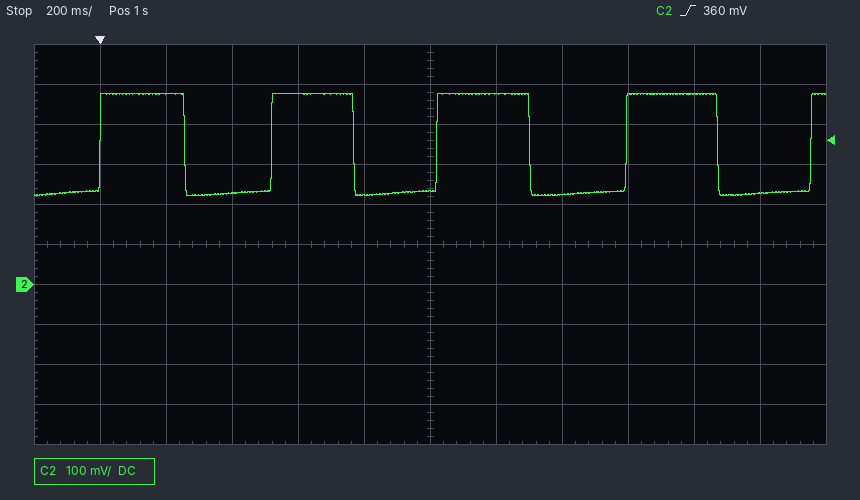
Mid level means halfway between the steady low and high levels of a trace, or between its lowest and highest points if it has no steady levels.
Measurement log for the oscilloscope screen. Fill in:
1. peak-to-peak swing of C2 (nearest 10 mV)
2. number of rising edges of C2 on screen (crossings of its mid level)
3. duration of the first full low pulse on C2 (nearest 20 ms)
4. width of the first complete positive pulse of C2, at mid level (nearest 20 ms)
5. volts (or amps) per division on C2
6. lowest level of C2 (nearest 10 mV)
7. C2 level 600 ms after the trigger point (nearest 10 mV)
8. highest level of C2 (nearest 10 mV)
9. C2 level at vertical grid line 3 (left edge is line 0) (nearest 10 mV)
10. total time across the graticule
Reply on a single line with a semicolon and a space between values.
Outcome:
260 mV; 5; 260 ms; 260 ms; 100 mV; 220 mV; 480 mV; 480 mV; 230 mV; 2.4 s
